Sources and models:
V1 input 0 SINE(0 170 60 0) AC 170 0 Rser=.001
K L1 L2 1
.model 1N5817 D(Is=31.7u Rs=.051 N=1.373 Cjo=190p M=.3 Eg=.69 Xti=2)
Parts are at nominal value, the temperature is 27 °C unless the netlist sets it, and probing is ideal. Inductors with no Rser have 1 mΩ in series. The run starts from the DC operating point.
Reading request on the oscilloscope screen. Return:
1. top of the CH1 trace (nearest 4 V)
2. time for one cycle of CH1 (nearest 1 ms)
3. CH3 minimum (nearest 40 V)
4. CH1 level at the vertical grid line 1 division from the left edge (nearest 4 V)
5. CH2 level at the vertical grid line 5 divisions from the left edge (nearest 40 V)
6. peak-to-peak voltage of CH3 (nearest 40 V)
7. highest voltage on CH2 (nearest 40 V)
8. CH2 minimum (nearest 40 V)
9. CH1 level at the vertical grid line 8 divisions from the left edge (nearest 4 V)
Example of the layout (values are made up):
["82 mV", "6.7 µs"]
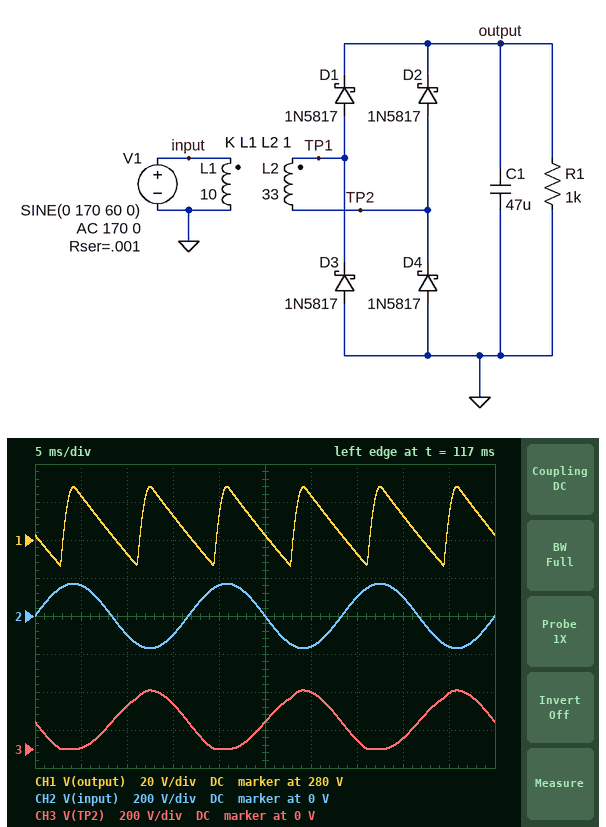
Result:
["308 V", "8 ms", "0 V", "304 V", "0 V", "320 V", "160 V", "-160 V", "292 V"]
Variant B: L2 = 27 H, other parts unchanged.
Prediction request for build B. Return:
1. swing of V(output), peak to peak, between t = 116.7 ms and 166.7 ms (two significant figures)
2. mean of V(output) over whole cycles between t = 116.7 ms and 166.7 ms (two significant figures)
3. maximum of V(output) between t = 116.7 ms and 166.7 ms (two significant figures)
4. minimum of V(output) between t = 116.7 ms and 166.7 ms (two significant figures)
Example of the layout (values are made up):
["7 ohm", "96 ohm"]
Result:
["38 V", "260 V", "280 V", "240 V"]
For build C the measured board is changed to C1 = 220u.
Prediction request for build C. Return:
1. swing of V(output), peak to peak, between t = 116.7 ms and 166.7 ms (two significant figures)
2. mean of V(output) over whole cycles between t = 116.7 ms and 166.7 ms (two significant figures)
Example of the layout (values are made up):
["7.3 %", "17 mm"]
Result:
["10 V", "300 V"]
